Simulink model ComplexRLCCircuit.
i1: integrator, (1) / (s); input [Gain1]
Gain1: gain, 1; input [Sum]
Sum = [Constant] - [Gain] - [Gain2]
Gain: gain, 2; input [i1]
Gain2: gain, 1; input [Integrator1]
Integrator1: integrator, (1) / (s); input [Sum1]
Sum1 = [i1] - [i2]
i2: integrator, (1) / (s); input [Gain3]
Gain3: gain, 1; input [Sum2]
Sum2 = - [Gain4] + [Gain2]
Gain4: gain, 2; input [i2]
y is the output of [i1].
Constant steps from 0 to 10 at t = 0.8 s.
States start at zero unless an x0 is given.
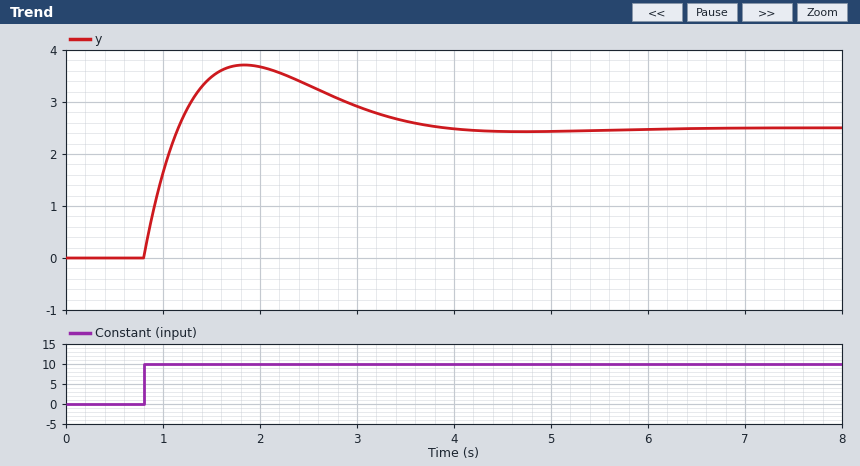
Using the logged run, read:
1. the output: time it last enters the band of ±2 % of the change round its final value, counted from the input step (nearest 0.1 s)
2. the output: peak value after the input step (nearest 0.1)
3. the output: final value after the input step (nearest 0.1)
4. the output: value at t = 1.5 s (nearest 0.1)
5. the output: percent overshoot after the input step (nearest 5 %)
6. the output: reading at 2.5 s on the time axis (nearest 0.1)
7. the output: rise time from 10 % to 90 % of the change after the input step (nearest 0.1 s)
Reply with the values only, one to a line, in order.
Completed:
4.6 s
3.7
2.5
3.5
50 %
3.3
0.3 s
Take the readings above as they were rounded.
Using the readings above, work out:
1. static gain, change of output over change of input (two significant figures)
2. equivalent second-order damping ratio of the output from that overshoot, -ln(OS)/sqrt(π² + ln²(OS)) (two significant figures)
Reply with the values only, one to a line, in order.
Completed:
0.25
0.22
